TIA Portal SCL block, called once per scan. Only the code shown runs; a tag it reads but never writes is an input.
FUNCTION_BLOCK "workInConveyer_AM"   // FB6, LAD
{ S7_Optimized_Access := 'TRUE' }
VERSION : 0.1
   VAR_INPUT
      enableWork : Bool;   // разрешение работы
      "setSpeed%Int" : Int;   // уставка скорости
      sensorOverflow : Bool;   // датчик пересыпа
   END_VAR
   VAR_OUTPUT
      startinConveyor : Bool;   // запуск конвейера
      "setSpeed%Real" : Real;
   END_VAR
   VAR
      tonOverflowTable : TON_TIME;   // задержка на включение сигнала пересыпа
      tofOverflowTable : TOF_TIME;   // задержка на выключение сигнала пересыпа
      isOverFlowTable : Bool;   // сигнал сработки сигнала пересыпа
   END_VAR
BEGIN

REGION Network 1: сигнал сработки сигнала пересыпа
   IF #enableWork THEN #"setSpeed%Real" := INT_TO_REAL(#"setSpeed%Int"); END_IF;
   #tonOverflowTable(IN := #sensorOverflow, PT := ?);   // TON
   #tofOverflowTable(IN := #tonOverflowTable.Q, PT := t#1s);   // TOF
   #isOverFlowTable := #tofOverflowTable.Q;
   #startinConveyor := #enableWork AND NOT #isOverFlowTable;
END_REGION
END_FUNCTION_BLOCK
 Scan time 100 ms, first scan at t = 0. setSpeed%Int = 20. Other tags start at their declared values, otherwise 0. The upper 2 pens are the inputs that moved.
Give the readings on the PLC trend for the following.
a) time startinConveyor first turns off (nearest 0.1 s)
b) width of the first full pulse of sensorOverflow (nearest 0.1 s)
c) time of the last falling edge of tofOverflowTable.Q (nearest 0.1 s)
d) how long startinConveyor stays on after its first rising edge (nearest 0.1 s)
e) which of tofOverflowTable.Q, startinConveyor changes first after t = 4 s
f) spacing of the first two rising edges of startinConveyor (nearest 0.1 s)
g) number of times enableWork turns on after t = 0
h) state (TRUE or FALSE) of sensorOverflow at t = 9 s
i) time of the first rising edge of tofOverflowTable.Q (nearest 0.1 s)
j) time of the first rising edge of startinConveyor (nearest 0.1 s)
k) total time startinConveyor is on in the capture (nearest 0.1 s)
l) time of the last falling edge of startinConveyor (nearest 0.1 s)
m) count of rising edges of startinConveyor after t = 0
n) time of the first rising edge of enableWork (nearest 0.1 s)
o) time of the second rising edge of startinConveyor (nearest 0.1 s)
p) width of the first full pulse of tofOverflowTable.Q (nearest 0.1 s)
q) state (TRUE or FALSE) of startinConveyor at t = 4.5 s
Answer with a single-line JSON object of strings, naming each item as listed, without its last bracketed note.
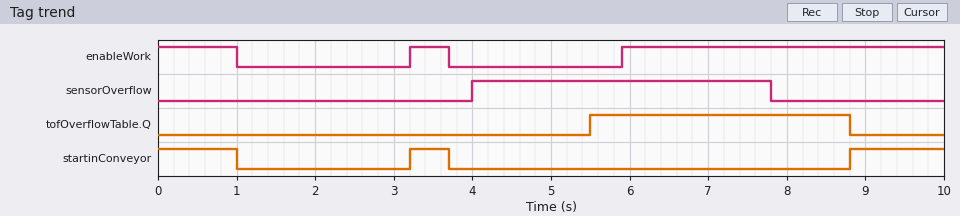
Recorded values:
{"time startinConveyor first turns off": "1.0 s", "width of the first full pulse of sensorOverflow": "3.8 s", "time of the last falling edge of tofOverflowTable.Q": "8.8 s", "how long startinConveyor stays on after its first rising edge": "0.5 s", "which of tofOverflowTable.Q, startinConveyor changes first after t = 4 s": "tofOverflowTable.Q", "spacing of the first two rising edges of startinConveyor": "5.6 s", "number of times enableWork turns on after t = 0": "2", "state (TRUE or FALSE) of sensorOverflow at t = 9 s": "FALSE", "time of the first rising edge of tofOverflowTable.Q": "5.5 s", "time of the first rising edge of startinConveyor": "3.2 s", "total time startinConveyor is on in the capture": "2.7 s", "time of the last falling edge of startinConveyor": "3.7 s", "count of rising edges of startinConveyor after t = 0": "2", "time of the first rising edge of enableWork": "3.2 s", "time of the second rising edge of startinConveyor": "8.8 s", "width of the first full pulse of tofOverflowTable.Q": "3.3 s", "state (TRUE or FALSE) of startinConveyor at t = 4.5 s": "FALSE"}
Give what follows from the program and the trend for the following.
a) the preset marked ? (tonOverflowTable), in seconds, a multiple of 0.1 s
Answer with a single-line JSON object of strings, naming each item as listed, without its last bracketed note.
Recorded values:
{"the preset marked ? (tonOverflowTable), in seconds, a multiple of 0.1 s": "1.5 s"}
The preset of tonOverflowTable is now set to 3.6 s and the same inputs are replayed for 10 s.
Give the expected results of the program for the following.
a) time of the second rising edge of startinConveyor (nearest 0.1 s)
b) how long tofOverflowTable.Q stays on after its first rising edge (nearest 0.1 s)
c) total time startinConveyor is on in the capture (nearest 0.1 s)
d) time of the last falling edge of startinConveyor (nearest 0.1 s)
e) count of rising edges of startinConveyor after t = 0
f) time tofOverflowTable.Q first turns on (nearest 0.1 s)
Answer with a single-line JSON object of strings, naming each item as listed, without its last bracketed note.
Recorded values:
{"time of the second rising edge of startinConveyor": "5.9 s", "how long tofOverflowTable.Q stays on after its first rising edge": "1.2 s", "total time startinConveyor is on in the capture": "4.4 s", "time of the last falling edge of startinConveyor": "7.6 s", "count of rising edges of startinConveyor after t = 0": "3", "time tofOverflowTable.Q first turns on": "7.6 s"}
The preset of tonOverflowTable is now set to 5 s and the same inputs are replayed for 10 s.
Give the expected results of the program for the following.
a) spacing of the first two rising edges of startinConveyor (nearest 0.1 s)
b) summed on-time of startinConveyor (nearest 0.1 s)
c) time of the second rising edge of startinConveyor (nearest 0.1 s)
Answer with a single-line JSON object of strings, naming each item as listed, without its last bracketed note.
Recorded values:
{"spacing of the first two rising edges of startinConveyor": "2.7 s", "summed on-time of startinConveyor": "5.6 s", "time of the second rising edge of startinConveyor": "5.9 s"}
